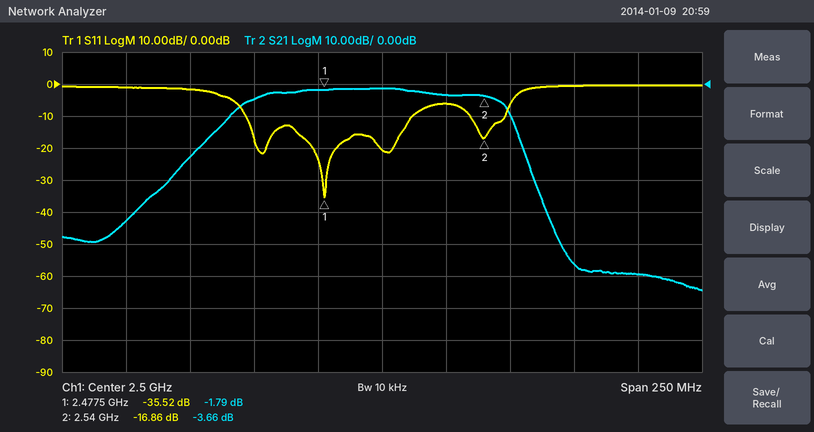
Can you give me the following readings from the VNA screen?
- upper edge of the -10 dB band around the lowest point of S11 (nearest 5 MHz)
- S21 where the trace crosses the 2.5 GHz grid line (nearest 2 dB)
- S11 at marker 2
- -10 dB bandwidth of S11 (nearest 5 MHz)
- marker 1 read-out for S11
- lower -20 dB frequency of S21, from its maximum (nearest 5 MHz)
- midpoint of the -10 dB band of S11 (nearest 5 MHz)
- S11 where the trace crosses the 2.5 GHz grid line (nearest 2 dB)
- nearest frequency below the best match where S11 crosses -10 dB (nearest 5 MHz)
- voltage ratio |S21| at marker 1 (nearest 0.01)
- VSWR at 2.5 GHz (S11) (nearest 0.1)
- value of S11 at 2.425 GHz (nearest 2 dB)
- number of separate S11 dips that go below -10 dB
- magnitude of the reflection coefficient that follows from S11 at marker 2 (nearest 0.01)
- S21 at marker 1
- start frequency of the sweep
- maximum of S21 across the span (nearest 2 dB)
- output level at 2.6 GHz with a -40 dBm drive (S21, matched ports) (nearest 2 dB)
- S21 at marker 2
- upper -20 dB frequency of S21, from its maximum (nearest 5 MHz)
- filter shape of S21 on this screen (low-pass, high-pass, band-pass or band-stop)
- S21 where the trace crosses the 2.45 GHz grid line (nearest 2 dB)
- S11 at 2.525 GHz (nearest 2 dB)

2.510 GHz
-2 dB
-16.86 dB
65 MHz
-35.52 dB
2.425 GHz
2.480 GHz
-20 dB
2.445 GHz
0.81
1.2
-2 dB
4
0.14
-1.79 dB
2.375 GHz
-2 dB
-100 dBm
-3.66 dB
2.555 GHz
band-pass
-4 dB
-6 dB
